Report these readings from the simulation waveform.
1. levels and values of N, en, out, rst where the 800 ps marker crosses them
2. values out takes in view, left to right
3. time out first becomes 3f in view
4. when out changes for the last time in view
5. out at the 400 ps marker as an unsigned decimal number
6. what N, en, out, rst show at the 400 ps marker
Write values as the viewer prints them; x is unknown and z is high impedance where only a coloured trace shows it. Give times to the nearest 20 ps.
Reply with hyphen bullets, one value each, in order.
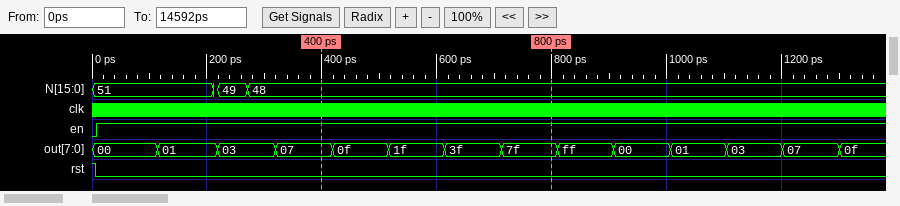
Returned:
- N=48, en=1, out=7f, rst=0
- 00, 01, 03, 07, 0f, 1f, 3f, 7f, ff, 00, 01, 03, 07, 0f
- 620 ps
- 1300 ps
- 7
- N=48, en=1, out=07, rst=0
